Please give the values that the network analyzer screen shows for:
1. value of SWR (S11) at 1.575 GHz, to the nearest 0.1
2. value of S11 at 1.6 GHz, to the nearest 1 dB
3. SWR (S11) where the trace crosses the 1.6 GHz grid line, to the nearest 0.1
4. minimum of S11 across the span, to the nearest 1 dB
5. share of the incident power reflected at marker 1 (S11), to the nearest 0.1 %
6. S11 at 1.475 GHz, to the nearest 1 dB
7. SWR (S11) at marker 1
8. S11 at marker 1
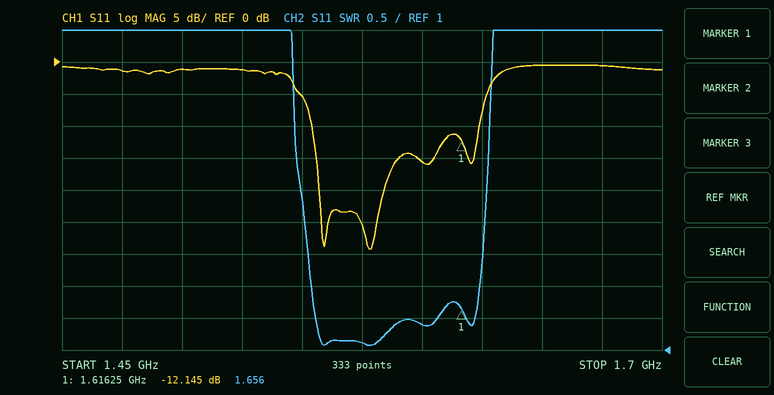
1.1
-16 dB
1.4
-29 dB
6.1 %
-1 dB
1.656
-12.145 dB
